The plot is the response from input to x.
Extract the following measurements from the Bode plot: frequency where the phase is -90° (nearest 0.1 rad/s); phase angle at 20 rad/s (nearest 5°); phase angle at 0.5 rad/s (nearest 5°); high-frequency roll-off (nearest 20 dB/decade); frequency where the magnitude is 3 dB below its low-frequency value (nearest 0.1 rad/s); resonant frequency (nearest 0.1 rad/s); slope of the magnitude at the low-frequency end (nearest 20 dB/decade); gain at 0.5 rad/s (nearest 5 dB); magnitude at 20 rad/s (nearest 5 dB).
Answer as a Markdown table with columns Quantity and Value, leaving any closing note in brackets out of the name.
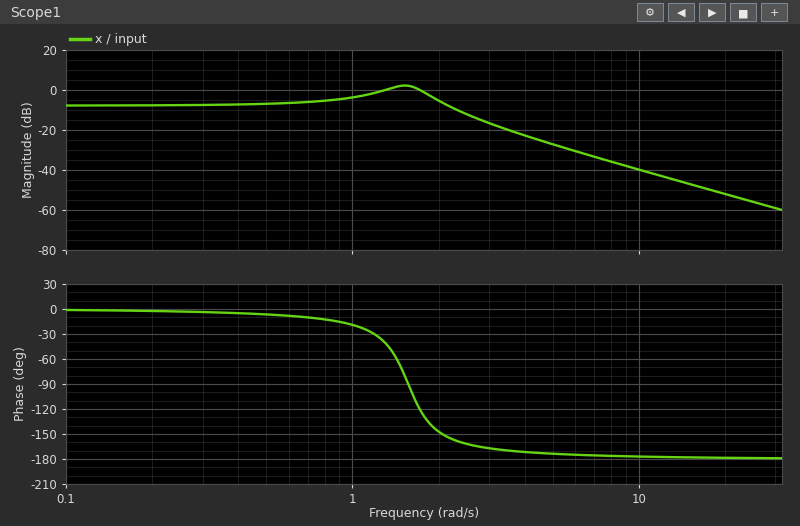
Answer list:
| Quantity | Value |
|---|---|
| frequency where the phase is -90° | 1.6 rad/s |
| phase angle at 20 rad/s | -180° |
| phase angle at 0.5 rad/s | -5° |
| high-frequency roll-off | -40 dB/decade |
| frequency where the magnitude is 3 dB below its low-frequency value | 2.4 rad/s |
| resonant frequency | 1.5 rad/s |
| slope of the magnitude at the low-frequency end | 0 dB/decade |
| gain at 0.5 rad/s | -5 dB |
| magnitude at 20 rad/s | -50 dB |
